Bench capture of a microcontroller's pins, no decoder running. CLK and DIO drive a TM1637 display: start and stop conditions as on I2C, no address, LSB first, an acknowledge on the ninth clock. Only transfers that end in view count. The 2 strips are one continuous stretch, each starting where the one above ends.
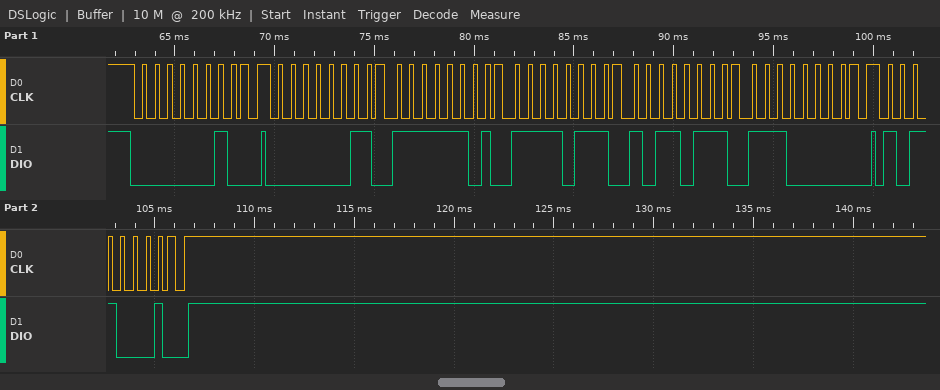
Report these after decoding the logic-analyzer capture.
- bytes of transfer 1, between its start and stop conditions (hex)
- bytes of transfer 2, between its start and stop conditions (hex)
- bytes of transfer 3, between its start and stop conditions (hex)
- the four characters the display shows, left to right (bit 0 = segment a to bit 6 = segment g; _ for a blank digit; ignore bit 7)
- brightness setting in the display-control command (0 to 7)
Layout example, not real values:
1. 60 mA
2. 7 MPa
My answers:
1. 40
2. C0 BF EF ED 07
3. 8D
4. 0957
5. 5
